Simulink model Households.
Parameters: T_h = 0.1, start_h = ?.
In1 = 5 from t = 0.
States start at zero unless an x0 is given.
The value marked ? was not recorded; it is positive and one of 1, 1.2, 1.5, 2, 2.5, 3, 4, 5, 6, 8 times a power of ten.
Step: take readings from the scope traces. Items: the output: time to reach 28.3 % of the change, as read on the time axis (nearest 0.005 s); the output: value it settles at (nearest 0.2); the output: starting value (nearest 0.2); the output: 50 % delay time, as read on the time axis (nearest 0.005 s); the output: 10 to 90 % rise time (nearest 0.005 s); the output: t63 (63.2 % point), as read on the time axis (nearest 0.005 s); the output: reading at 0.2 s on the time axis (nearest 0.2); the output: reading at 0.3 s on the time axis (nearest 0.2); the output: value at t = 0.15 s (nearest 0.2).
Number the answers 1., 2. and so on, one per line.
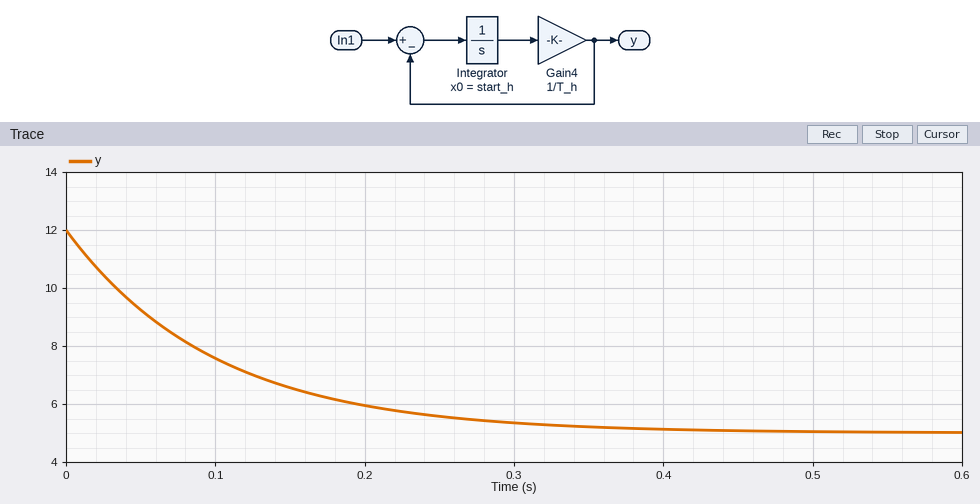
1. 0.035 s
2. 5.0
3. 12.0
4. 0.070 s
5. 0.220 s
6. 0.100 s
7. 6.0
8. 5.4
9. 6.6
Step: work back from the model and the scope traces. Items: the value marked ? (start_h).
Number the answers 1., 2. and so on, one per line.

1. 1.2
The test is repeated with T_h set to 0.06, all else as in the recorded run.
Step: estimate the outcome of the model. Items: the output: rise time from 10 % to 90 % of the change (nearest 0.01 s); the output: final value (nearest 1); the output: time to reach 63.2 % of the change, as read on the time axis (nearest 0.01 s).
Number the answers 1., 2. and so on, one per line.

1. 0.13 s
2. 5
3. 0.06 s
